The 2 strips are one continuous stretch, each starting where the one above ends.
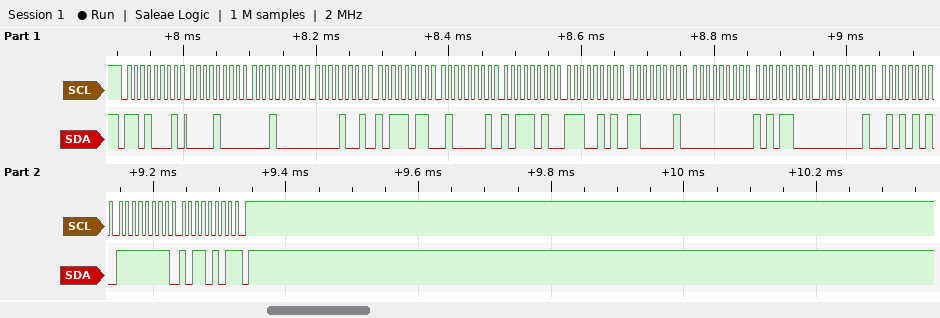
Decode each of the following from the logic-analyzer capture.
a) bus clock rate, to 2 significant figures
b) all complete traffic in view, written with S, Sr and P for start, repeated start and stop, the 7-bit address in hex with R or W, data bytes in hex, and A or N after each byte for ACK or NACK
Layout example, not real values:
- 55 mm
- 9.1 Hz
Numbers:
- 100 kHz
- S 68R A 08 A 10 A 09 A BB A 41 A BA A E5 A C1 A 00 A AC A 01 A 55 A FF A B5 N P
